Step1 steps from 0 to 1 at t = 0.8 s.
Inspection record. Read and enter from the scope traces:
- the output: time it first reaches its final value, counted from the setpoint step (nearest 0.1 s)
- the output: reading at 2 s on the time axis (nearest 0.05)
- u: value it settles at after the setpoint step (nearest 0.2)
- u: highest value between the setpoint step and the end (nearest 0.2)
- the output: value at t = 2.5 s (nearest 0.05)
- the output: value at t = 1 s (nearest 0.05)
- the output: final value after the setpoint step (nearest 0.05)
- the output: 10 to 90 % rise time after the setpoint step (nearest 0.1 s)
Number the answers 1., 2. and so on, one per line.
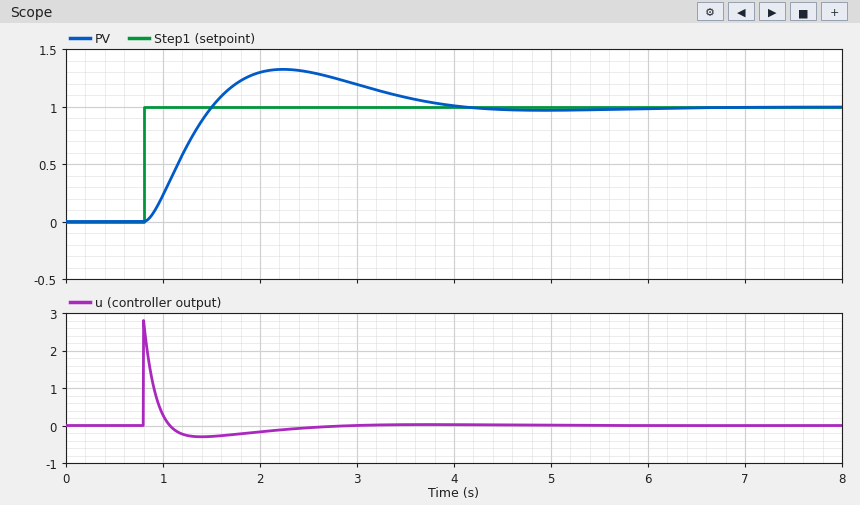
1. 0.7 s
2. 1.30
3. 0.0
4. 2.8
5. 1.30
6. 0.25
7. 1.00
8. 0.5 s
